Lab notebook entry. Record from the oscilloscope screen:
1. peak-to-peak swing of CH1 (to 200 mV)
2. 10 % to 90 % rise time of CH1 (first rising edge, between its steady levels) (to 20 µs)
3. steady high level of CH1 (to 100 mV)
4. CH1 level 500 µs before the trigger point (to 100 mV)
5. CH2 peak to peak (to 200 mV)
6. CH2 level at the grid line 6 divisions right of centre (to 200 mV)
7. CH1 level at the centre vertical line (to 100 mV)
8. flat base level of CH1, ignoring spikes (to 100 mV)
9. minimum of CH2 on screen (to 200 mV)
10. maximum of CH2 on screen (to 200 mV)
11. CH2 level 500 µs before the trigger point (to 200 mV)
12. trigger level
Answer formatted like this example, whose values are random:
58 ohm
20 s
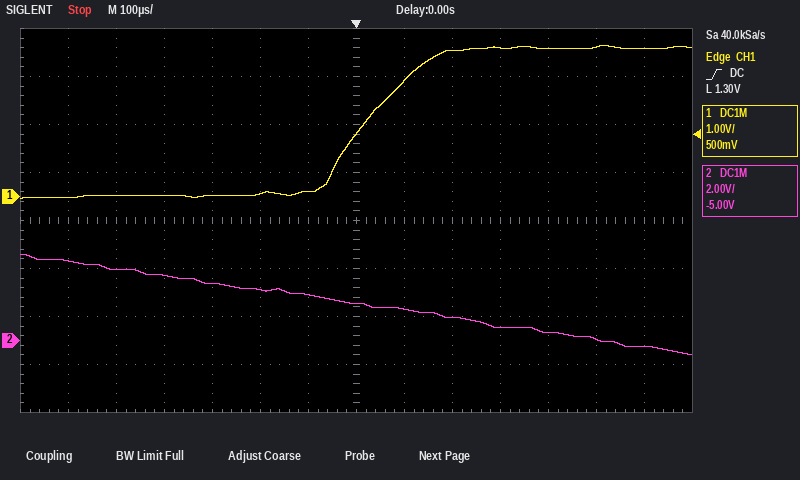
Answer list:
3.2 V
200 µs
3.1 V
0.0 V
4.2 V
-200 mV
1.3 V
0.0 V
-600 mV
3.6 V
3.0 V
1.30 V
